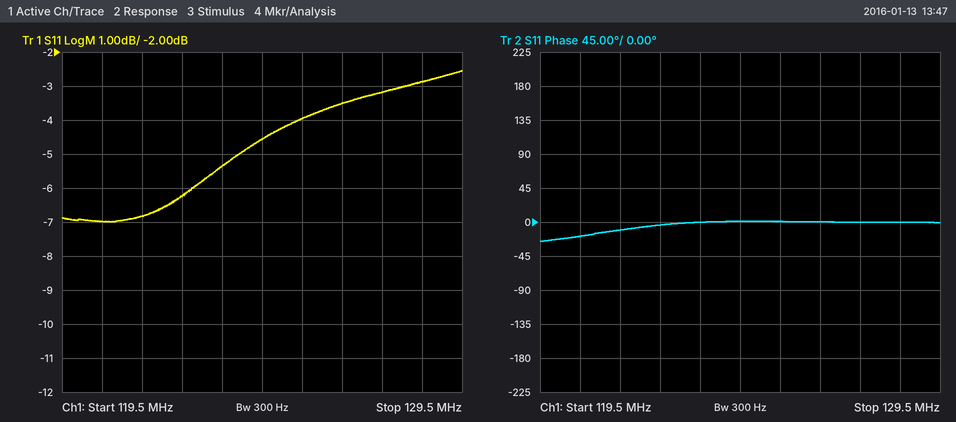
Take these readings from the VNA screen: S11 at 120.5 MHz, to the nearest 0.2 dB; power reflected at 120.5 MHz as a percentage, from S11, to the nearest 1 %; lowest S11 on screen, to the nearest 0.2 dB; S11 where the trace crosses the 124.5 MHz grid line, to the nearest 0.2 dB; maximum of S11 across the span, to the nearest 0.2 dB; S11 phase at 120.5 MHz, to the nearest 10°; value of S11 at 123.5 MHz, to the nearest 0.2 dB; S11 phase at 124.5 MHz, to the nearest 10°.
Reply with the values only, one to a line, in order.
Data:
-7.0 dB
20 %
-7.0 dB
-4.6 dB
-2.6 dB
-20°
-5.4 dB
0°
